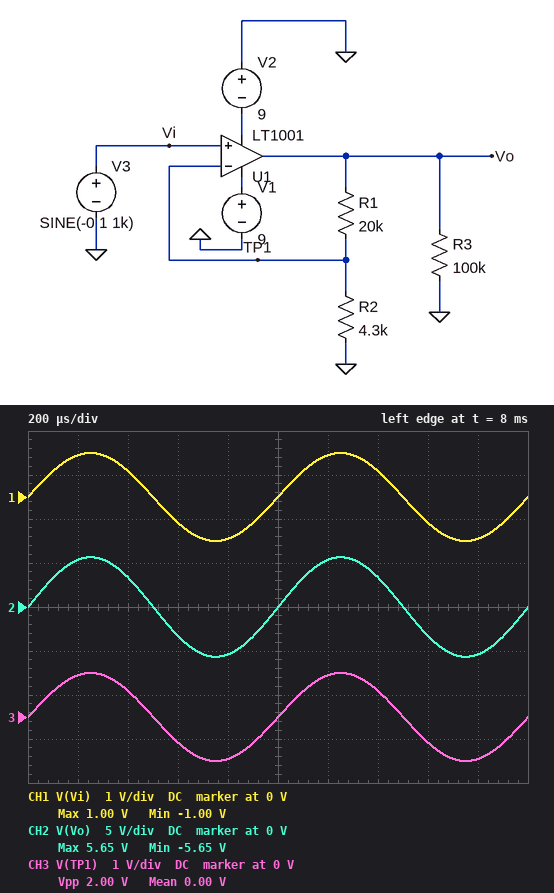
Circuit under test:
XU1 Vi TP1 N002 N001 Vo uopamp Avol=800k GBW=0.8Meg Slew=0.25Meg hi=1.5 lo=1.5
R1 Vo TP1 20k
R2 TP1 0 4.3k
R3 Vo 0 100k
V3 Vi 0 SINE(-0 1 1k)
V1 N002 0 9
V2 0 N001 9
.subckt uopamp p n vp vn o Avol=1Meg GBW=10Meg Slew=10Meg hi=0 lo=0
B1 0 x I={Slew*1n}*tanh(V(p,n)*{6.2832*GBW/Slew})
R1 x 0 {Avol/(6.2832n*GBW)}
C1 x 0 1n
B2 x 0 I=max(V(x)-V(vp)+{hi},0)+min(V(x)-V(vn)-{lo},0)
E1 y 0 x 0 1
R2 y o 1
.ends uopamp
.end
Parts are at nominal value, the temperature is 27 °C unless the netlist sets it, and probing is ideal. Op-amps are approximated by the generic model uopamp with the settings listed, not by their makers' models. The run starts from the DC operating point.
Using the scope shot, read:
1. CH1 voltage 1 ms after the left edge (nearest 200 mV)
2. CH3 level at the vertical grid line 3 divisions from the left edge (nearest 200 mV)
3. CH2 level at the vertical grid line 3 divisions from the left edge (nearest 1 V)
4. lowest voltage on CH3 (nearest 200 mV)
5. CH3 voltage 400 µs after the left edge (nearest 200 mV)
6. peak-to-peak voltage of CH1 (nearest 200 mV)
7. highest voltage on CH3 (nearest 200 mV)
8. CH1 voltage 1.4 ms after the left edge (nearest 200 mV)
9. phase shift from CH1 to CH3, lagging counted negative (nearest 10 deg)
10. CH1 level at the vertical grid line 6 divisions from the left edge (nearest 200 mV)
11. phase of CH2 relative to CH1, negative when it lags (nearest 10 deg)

0 V
-600 mV
-3 V
-1.0 V
600 mV
2.0 V
1.0 V
600 mV
0 deg
1.0 V
0 deg
